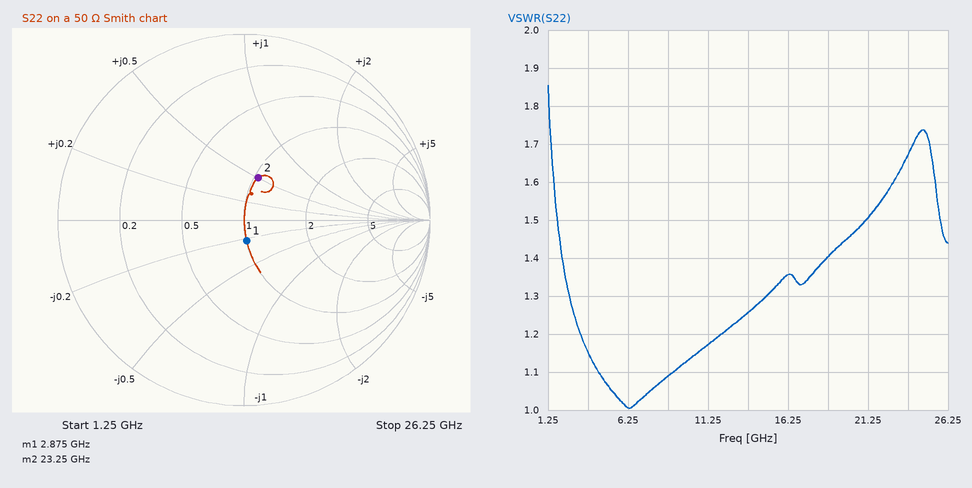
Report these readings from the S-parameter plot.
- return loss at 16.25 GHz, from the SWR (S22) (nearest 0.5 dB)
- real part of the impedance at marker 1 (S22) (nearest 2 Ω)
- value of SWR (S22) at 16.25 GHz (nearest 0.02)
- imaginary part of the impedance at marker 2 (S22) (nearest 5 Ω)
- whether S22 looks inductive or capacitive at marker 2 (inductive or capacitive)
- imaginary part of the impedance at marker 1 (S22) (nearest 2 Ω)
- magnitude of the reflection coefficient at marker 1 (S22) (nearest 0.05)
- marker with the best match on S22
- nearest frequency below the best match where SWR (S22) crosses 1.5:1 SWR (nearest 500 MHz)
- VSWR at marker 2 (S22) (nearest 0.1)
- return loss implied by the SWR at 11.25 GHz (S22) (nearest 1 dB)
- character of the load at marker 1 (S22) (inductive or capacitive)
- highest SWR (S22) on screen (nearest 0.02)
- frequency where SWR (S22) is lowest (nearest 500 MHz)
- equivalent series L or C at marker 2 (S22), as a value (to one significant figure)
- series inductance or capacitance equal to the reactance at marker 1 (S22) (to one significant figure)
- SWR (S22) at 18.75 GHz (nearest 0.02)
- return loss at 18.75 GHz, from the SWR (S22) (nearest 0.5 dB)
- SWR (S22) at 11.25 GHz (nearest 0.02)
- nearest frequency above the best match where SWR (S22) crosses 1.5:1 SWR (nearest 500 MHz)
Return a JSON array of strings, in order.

["16.5 dB", "50 Ω", "1.36", "+25 Ω", "inductive", "-12 Ω", "0.10", "marker 1", "2.0 GHz", "1.6", "22 dB", "capacitive", "1.86", "6.5 GHz", "200 pH", "5 pF", "1.40", "15.5 dB", "1.18", "21.0 GHz"]
